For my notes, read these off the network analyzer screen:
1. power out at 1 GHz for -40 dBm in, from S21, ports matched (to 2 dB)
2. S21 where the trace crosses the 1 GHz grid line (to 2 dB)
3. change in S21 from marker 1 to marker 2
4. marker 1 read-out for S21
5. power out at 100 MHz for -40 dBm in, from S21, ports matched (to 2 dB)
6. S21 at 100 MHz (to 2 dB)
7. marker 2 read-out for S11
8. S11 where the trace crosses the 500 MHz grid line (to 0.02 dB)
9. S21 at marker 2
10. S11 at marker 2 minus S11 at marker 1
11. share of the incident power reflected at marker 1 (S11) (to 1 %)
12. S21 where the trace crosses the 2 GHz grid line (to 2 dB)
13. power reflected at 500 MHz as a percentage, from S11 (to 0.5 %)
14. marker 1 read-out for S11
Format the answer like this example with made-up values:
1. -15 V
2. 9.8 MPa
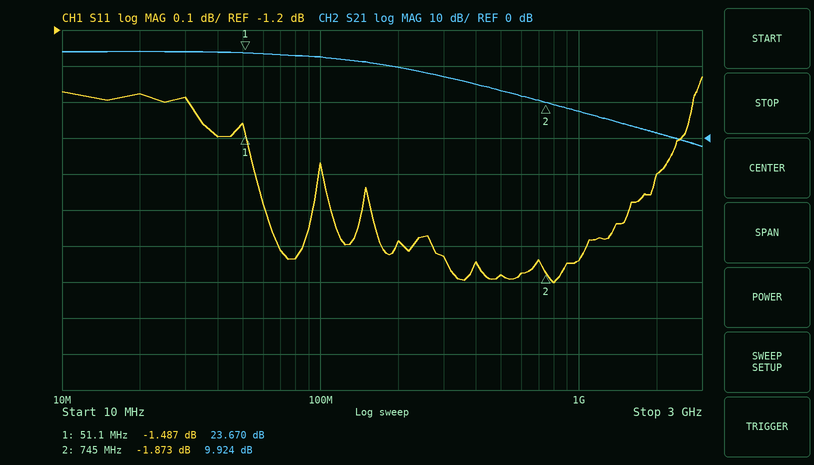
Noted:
1. -32 dBm
2. 8 dB
3. -13.746 dB
4. 23.670 dB
5. -18 dBm
6. 22 dB
7. -1.873 dB
8. -1.88 dB
9. 9.924 dB
10. -0.386 dB
11. 71 %
12. 2 dB
13. 65.0 %
14. -1.487 dB
